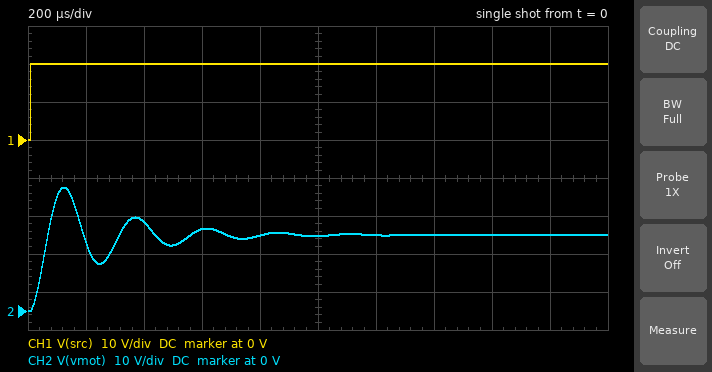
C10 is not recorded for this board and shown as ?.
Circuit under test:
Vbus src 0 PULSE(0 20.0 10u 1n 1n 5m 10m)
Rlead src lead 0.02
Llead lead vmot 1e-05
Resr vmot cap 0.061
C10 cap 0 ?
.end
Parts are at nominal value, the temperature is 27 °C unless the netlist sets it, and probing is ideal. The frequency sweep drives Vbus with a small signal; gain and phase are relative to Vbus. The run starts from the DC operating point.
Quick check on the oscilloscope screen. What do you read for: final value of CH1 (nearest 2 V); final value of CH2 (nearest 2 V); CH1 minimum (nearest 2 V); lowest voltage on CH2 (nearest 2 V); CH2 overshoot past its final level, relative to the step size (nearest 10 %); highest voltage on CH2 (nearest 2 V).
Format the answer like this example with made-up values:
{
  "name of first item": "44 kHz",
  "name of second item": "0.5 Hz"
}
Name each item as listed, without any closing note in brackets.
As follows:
{
  "final value of CH1": "20 V",
  "final value of CH2": "20 V",
  "CH1 minimum": "0 V",
  "lowest voltage on CH2": "0 V",
  "CH2 overshoot past its final level, relative to the step size": "60 %",
  "highest voltage on CH2": "32 V"
}
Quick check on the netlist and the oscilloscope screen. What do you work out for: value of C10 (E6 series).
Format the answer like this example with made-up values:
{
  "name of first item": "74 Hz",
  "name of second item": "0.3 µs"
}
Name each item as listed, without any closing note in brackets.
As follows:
{
  "value of C10": "150 µF"
}
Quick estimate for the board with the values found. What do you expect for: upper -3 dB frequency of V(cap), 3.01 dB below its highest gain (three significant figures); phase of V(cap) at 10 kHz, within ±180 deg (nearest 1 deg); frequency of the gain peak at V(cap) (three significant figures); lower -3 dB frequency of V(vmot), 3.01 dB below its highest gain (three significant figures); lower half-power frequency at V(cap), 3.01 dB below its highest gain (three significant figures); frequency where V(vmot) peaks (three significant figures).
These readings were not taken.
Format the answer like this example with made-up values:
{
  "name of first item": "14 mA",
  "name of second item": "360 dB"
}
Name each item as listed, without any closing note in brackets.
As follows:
{
  "upper -3 dB frequency of V(cap), 3.01 dB below its highest gain": "4.61 kHz",
  "phase of V(cap) at 10 kHz, within ±180 deg": "-171 deg",
  "frequency of the gain peak at V(cap)": "4.01 kHz",
  "lower -3 dB frequency of V(vmot), 3.01 dB below its highest gain": "3.30 kHz",
  "lower half-power frequency at V(cap), 3.01 dB below its highest gain": "3.29 kHz",
  "frequency where V(vmot) peaks": "4.01 kHz"
}
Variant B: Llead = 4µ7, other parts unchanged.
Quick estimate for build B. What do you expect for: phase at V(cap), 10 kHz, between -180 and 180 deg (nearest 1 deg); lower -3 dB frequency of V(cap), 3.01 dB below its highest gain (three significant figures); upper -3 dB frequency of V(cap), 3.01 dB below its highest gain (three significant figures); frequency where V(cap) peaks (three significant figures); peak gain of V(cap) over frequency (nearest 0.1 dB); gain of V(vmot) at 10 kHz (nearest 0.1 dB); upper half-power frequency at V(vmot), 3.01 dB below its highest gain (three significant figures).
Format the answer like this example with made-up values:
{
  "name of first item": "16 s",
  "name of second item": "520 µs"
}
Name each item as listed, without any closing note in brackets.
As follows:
{
  "phase at V(cap), 10 kHz, between -180 and 180 deg": "-157 deg",
  "lower -3 dB frequency of V(cap), 3.01 dB below its highest gain": "4.02 kHz",
  "upper -3 dB frequency of V(cap), 3.01 dB below its highest gain": "6.94 kHz",
  "frequency where V(cap) peaks": "5.67 kHz",
  "peak gain of V(cap) over frequency": "7.0 dB",
  "gain of V(vmot) at 10 kHz": "-4.5 dB",
  "upper half-power frequency at V(vmot), 3.01 dB below its highest gain": "7.00 kHz"
}
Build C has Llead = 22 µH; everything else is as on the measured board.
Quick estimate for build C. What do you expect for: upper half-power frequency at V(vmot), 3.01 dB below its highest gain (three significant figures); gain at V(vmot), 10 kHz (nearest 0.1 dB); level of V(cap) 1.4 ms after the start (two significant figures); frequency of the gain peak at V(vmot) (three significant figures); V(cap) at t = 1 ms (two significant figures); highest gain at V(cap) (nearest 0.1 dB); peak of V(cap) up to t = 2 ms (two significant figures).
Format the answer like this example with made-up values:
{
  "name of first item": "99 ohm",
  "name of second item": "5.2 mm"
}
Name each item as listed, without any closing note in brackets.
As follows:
{
  "upper half-power frequency at V(vmot), 3.01 dB below its highest gain": "3.02 kHz",
  "gain at V(vmot), 10 kHz": "-20.4 dB",
  "level of V(cap) 1.4 ms after the start": "19 V",
  "frequency of the gain peak at V(vmot)": "2.74 kHz",
  "V(cap) at t = 1 ms": "21 V",
  "highest gain at V(cap)": "13.5 dB",
  "peak of V(cap) up to t = 2 ms": "34 V"
}
